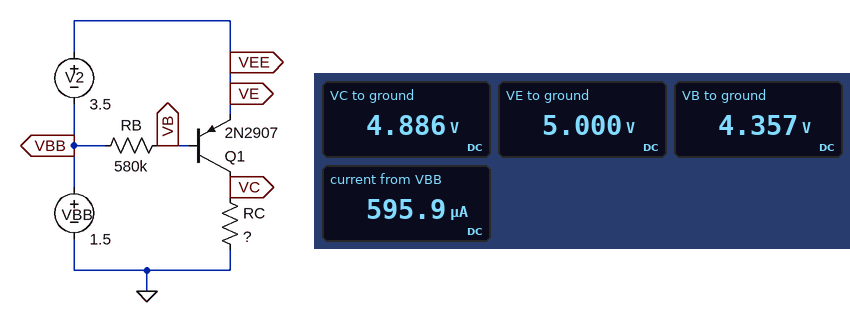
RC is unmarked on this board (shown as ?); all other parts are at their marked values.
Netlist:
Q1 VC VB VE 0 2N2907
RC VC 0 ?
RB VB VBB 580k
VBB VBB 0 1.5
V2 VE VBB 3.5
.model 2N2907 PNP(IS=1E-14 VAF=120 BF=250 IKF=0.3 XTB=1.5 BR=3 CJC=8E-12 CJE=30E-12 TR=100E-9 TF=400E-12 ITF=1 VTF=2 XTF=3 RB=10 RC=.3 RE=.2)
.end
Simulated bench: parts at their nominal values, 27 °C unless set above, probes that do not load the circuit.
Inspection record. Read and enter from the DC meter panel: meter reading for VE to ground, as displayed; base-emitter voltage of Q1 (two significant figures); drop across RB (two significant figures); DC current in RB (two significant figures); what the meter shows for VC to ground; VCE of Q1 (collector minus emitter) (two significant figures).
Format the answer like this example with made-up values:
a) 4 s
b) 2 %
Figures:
a) 5.000 V
b) -640 mV
c) 2.9 V
d) 4.9 µA
e) 4.886 V
f) -110 mV
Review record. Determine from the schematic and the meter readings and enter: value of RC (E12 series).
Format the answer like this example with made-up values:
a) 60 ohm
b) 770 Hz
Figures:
a) 8.2 kΩ
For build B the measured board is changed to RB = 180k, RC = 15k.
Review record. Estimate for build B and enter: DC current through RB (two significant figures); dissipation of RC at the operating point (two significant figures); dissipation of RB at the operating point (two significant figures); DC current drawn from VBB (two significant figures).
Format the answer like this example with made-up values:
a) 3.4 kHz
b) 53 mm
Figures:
a) 16 µA
b) 1.6 mW
c) 46 µW
d) 330 µA
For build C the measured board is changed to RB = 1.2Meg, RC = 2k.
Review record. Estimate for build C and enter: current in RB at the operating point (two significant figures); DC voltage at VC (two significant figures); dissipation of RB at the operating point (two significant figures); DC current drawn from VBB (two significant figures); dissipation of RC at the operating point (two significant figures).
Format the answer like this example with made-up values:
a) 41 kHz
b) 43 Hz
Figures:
a) 2.4 µA
b) 1.2 V
c) 6.8 µW
d) 610 µA
e) 740 µW
